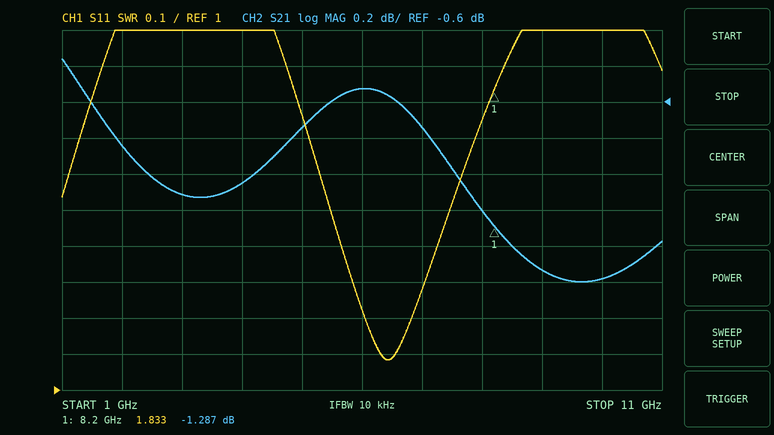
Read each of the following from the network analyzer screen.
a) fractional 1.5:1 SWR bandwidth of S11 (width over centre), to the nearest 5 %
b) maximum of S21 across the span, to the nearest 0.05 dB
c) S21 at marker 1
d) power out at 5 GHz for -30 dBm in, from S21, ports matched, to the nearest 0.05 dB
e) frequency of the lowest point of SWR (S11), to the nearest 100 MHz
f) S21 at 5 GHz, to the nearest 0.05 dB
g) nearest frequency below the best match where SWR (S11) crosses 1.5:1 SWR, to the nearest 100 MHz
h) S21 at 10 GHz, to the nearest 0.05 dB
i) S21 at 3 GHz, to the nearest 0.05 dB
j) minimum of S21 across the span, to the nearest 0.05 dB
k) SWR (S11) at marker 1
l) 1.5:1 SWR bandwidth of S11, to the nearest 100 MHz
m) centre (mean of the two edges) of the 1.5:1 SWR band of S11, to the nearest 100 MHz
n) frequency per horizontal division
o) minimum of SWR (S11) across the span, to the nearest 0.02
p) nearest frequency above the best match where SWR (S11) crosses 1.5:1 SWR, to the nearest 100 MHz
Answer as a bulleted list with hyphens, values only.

- 30 %
- -0.35 dB
- -1.287 dB
- -30.75 dBm
- 6.4 GHz
- -0.75 dB
- 5.5 GHz
- -1.60 dB
- -1.10 dB
- -1.60 dB
- 1.833
- 2.0 GHz
- 6.5 GHz
- 1 GHz
- 1.08
- 7.5 GHz
